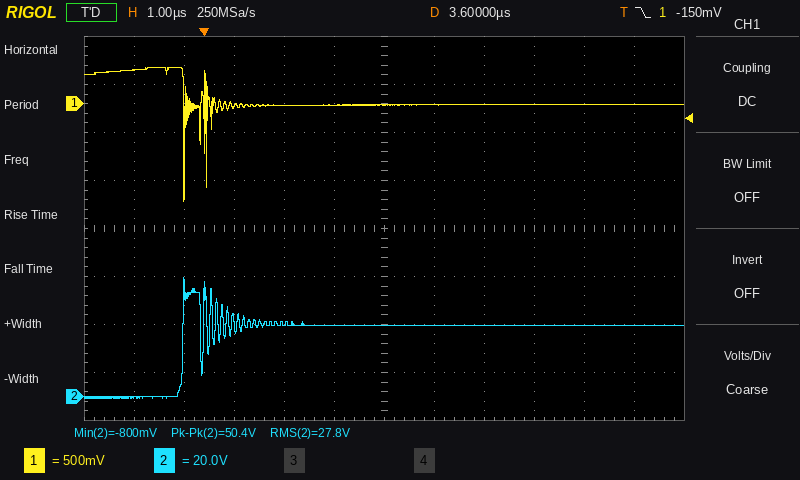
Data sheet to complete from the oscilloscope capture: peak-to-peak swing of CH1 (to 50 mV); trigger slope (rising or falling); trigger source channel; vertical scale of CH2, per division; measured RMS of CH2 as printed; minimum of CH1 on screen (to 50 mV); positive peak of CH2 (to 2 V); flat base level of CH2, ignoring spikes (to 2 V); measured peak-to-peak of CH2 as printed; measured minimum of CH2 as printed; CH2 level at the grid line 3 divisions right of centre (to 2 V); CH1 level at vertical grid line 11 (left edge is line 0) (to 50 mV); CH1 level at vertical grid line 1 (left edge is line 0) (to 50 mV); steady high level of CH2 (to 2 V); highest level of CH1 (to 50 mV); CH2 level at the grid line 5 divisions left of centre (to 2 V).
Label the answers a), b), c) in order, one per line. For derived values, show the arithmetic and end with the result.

a) 400 mV − (-1.00 V) = 1.40 V
b) falling
c) CH1
d) 20 V
e) 27.8 V
f) -1.00 V
g) 50 V
h) 0 V
i) 50.4 V
j) -800 mV
k) 30 V
l) 0 mV
m) 350 mV
n) 30 V
o) 400 mV
p) 0 V
